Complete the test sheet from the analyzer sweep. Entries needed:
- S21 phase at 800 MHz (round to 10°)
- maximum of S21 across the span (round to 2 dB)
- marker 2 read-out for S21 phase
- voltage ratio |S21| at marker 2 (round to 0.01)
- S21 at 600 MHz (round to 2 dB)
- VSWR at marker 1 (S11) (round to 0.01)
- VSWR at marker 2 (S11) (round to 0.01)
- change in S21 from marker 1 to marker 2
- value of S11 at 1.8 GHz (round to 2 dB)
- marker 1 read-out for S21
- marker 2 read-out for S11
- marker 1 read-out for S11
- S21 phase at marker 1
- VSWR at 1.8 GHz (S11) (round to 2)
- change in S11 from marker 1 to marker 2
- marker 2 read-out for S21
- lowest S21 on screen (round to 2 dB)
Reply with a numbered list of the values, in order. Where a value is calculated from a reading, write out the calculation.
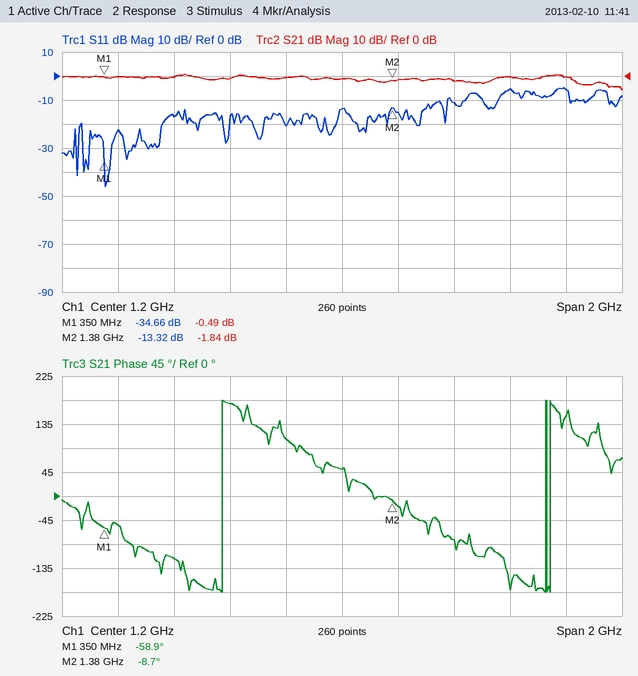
1. 170°
2. 0 dB
3. -8.7°
4. 10^(-1.84/20) ≈ 0.81
5. 0 dB
6. (1 + 0.0185)/(1 − 0.0185) ≈ 1.04
7. (1 + 0.2158)/(1 − 0.2158) ≈ 1.55
8. -1.84 − (-0.49) = -1.35 dB
9. -6 dB
10. -0.49 dB
11. -13.32 dB
12. -34.66 dB
13. -58.9°
14. |Γ| = 10^(-6/20) = 0.5012; VSWR = (1 + 0.5012)/(1 − 0.5012) ≈ 3.01, so 4 to the nearest 2
15. -13.32 − (-34.66) = 21.34 dB
16. -1.84 dB
17. -6 dB
